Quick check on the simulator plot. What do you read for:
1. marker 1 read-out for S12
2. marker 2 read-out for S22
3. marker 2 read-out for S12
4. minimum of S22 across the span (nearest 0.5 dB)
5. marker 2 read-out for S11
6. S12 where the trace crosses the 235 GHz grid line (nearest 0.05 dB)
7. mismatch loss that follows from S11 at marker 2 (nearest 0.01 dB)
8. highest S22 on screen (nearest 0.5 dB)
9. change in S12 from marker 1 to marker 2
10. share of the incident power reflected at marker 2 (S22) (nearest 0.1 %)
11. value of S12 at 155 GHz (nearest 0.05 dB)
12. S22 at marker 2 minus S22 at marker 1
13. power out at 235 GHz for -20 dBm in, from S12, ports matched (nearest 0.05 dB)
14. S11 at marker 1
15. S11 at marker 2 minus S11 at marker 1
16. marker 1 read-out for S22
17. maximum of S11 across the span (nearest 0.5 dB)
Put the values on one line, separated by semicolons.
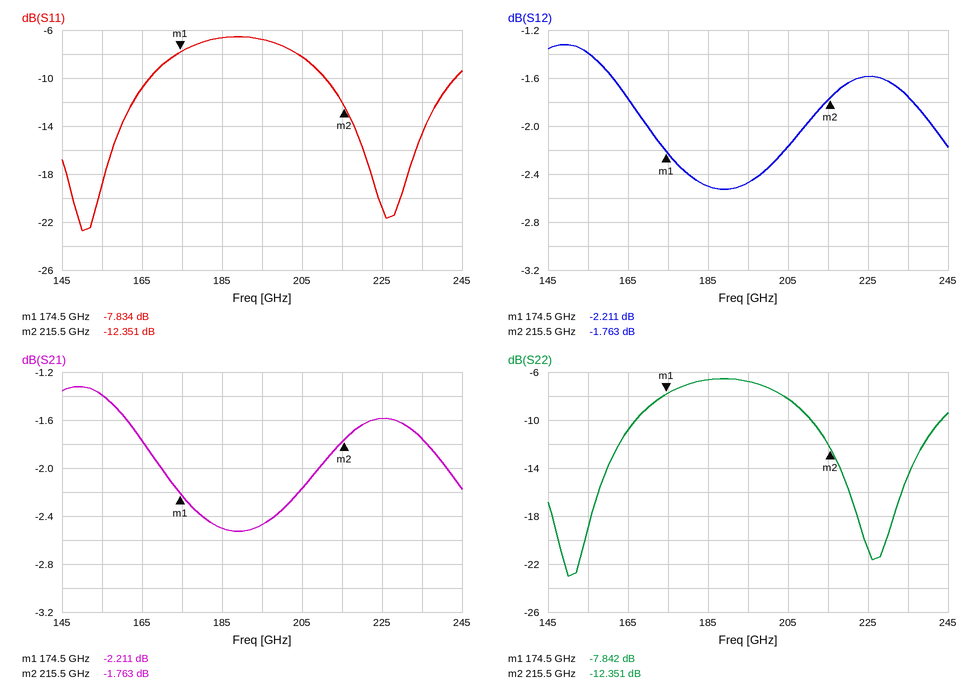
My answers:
-2.211 dB; -12.351 dB; -1.763 dB; -23.0 dB; -12.351 dB; -1.75 dB; 0.26 dB; -6.5 dB; 0.448 dB; 5.8 %; -1.40 dB; -4.509 dB; -21.75 dBm; -7.834 dB; -4.517 dB; -7.842 dB; -6.5 dB
